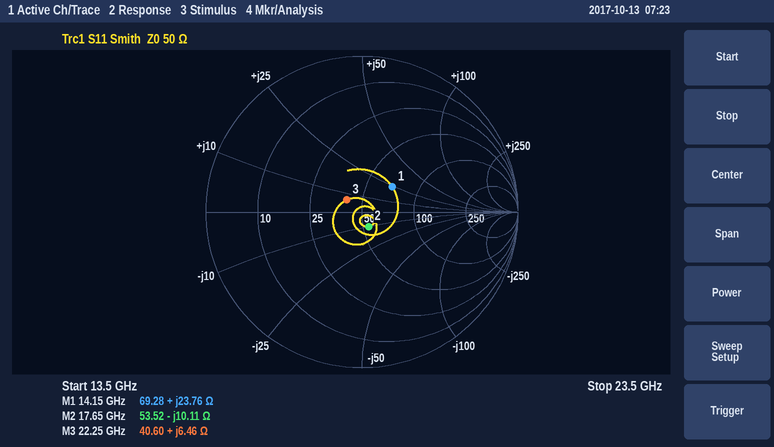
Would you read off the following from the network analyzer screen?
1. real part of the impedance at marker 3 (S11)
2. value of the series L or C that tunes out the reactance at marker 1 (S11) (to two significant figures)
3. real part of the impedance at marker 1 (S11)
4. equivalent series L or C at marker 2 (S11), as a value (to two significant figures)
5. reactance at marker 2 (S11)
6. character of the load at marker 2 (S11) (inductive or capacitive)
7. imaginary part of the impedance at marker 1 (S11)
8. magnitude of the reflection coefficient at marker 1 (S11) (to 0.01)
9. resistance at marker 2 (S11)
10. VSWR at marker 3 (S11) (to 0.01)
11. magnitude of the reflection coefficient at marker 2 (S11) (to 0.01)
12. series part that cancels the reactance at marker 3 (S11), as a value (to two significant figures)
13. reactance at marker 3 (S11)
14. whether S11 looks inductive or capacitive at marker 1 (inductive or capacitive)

40.60 Ω
470 fF
69.28 Ω
890 fF
-10.11 Ω
capacitive
+23.76 Ω
0.25
53.52 Ω
1.29
0.10
1.1 pF
+6.46 Ω
inductive
